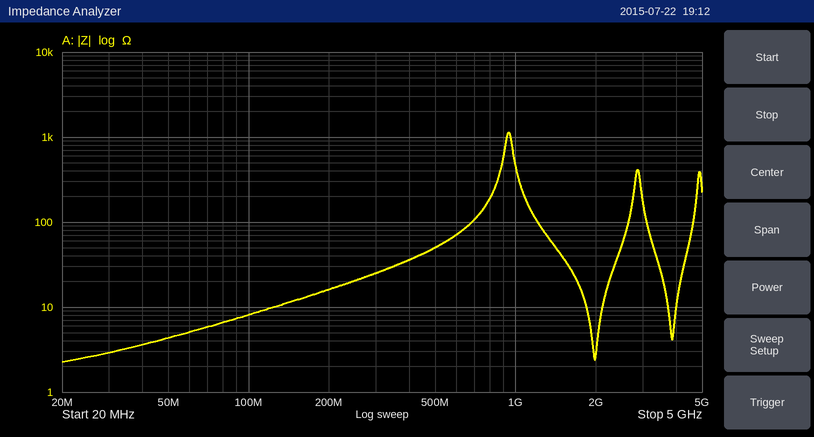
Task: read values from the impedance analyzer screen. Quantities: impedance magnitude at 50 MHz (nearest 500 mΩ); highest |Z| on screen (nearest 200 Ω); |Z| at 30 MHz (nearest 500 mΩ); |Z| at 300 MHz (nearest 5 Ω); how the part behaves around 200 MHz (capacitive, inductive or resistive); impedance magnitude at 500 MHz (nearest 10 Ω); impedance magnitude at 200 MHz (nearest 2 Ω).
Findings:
4.5 Ω
1.2 kΩ
3.0 Ω
25 Ω
inductive
50 Ω
16 Ω
